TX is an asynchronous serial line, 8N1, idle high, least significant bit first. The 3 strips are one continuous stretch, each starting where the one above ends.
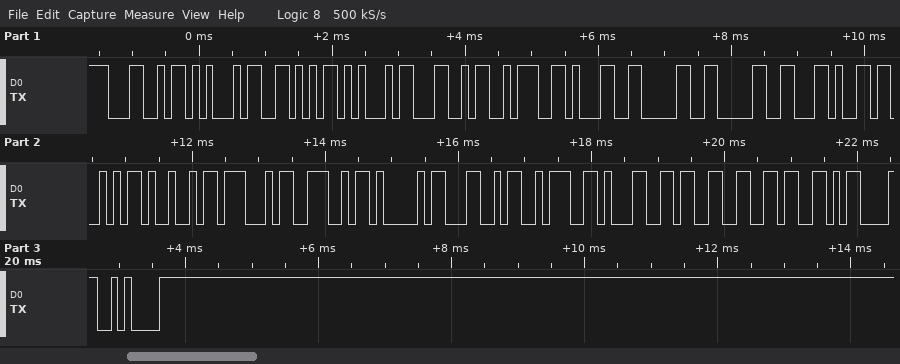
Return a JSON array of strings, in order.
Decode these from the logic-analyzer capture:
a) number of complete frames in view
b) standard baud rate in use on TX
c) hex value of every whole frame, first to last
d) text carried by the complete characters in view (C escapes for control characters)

["22", "9600 baud", "4C 45 56 45 4C 3A 31 30 30 2C 53 49 47 4E 41 4C 3A 31 33 36 0D 0A", "\"LEVEL:100,SIGNAL:136\\r\\n\""]
